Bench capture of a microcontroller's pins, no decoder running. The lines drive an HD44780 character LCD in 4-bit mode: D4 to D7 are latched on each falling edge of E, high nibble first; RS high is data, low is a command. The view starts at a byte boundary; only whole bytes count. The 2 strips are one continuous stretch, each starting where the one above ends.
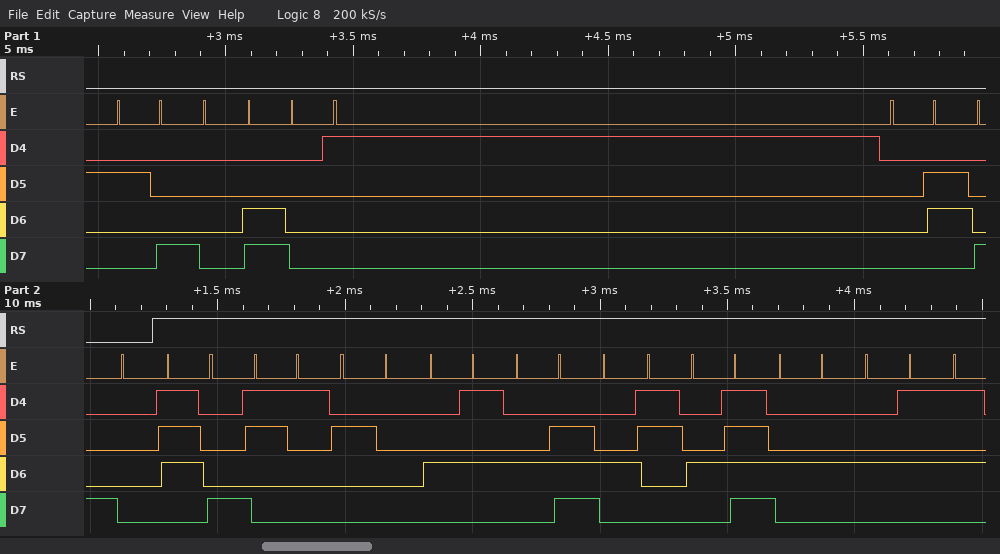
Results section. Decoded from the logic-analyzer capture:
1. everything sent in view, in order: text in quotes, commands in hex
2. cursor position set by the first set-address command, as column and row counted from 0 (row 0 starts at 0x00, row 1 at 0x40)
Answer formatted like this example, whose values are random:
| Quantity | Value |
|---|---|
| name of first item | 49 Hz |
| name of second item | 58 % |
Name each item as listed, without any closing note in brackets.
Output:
| Quantity | Value |
|---|---|
| everything sent in view, in order: text in quotes, commands in hex | 0x28 0x0C 0x01 0x06 0x80 "x1 ENCODE" |
| cursor position set by the first set-address command, as column and row counted from 0 | column 0, row 0 |
